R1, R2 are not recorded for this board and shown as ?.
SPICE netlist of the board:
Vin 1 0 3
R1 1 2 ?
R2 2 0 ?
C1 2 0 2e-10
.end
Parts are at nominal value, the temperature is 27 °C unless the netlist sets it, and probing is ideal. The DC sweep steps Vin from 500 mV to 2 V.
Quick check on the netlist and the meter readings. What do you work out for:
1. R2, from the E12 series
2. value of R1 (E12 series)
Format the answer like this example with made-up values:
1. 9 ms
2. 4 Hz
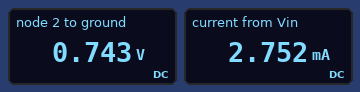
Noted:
1. 270 Ω
2. 820 Ω
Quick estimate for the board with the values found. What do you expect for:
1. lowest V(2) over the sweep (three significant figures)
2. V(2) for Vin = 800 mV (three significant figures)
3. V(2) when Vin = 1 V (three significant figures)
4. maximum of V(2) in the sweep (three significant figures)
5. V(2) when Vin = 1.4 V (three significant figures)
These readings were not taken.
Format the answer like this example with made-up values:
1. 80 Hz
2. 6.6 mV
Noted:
1. 124 mV
2. 198 mV
3. 248 mV
4. 495 mV
5. 347 mV
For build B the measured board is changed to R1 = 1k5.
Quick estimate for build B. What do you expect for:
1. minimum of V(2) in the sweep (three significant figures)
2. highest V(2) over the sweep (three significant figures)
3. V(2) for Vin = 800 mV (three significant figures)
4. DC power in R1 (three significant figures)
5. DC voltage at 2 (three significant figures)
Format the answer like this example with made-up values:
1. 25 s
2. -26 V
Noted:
1. 76.3 mV
2. 305 mV
3. 122 mV
4. 4.31 mW
5. 458 mV
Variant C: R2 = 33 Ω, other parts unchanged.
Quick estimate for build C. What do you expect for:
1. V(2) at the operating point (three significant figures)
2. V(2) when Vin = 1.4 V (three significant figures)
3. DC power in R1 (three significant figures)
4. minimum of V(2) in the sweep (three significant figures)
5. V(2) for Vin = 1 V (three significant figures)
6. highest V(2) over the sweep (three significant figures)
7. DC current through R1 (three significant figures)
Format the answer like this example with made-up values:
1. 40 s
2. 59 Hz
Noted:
1. 116 mV
2. 54.2 mV
3. 10.1 mW
4. 19.3 mV
5. 38.7 mV
6. 77.4 mV
7. 3.52 mA
